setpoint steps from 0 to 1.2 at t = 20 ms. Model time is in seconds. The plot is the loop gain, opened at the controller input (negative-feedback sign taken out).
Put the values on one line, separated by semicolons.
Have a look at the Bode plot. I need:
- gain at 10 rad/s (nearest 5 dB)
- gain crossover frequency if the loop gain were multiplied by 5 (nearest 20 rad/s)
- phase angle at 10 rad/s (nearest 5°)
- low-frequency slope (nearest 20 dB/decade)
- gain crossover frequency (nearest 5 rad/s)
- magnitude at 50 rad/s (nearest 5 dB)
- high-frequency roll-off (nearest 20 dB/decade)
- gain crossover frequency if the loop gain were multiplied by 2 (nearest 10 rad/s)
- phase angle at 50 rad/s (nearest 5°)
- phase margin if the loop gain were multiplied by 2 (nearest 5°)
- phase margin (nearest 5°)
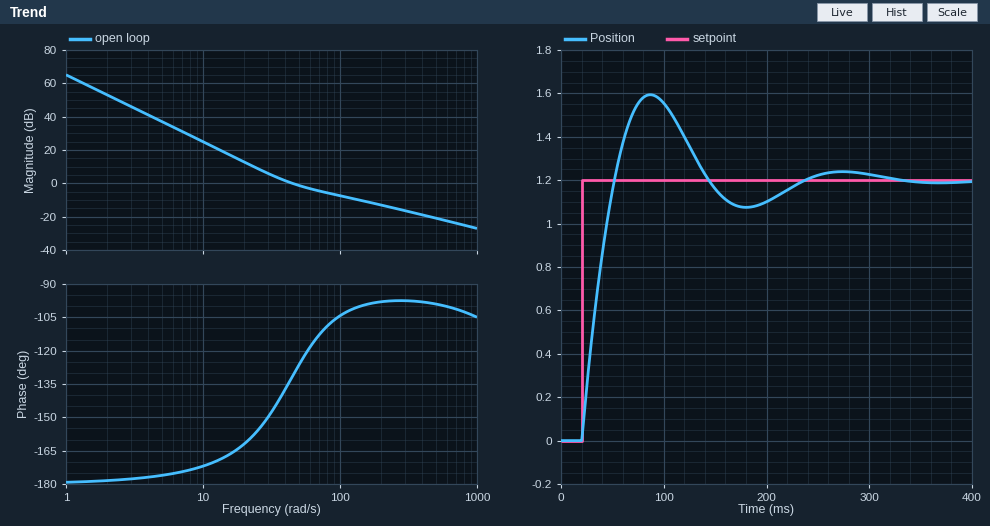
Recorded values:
25 dB; 220 rad/s; -170°; -40 dB/decade; 45 rad/s; 0 dB; -20 dB/decade; 80 rad/s; -125°; 70°; 50°
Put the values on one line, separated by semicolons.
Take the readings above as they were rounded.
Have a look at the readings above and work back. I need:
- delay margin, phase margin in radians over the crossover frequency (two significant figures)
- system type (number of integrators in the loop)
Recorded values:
0.019 s; 2
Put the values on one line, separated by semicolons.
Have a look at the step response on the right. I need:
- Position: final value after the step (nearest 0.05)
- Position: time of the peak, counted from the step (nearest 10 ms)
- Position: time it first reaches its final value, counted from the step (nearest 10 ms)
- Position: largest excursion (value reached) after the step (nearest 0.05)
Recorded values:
1.20; 70 ms; 30 ms; 1.60
